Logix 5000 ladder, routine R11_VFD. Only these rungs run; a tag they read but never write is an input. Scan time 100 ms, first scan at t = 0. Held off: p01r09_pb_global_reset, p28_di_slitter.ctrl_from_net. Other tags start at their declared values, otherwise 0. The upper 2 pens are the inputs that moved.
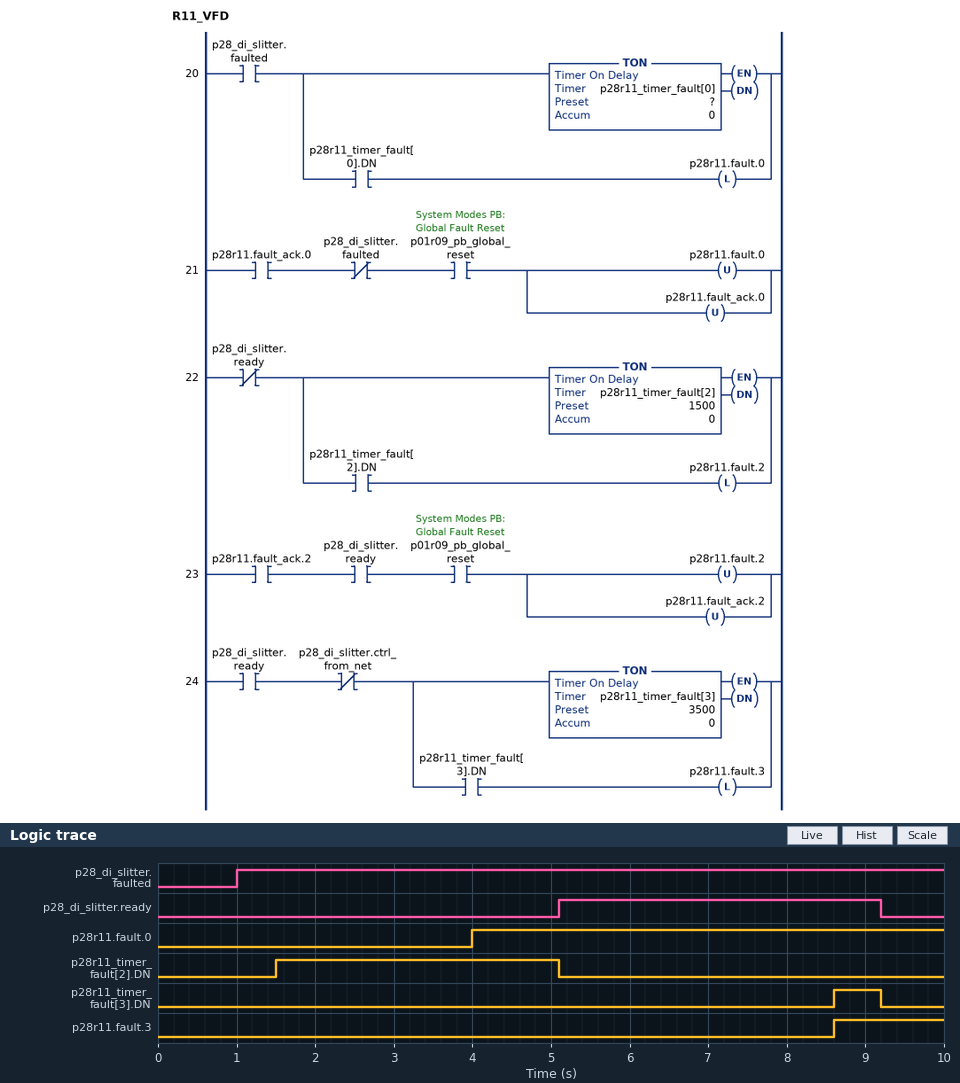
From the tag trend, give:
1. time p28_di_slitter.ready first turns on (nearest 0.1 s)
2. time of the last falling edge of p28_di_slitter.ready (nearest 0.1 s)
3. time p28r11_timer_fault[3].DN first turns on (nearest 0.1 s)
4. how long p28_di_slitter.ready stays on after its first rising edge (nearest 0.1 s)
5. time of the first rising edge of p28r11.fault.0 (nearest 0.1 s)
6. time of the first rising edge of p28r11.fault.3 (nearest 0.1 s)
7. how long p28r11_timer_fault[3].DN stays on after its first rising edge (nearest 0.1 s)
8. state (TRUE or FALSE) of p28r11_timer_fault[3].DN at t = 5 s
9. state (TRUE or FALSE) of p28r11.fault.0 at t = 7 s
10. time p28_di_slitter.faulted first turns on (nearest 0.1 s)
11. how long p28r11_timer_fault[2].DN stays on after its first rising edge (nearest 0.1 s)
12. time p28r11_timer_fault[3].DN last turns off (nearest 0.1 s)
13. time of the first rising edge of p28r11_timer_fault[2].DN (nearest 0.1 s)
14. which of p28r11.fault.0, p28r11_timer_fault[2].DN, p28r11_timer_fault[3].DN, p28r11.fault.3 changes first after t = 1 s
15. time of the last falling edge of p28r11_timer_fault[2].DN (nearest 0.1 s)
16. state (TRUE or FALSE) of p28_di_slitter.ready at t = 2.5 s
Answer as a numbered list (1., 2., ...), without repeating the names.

1. 5.1 s
2. 9.2 s
3. 8.6 s
4. 4.1 s
5. 4.0 s
6. 8.6 s
7. 0.6 s
8. FALSE
9. TRUE
10. 1.0 s
11. 3.6 s
12. 9.2 s
13. 1.5 s
14. p28r11_timer_fault[2].DN
15. 5.1 s
16. FALSE
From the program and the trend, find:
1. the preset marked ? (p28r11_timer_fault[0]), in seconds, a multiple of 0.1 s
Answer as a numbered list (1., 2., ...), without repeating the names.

1. 3.0 s
